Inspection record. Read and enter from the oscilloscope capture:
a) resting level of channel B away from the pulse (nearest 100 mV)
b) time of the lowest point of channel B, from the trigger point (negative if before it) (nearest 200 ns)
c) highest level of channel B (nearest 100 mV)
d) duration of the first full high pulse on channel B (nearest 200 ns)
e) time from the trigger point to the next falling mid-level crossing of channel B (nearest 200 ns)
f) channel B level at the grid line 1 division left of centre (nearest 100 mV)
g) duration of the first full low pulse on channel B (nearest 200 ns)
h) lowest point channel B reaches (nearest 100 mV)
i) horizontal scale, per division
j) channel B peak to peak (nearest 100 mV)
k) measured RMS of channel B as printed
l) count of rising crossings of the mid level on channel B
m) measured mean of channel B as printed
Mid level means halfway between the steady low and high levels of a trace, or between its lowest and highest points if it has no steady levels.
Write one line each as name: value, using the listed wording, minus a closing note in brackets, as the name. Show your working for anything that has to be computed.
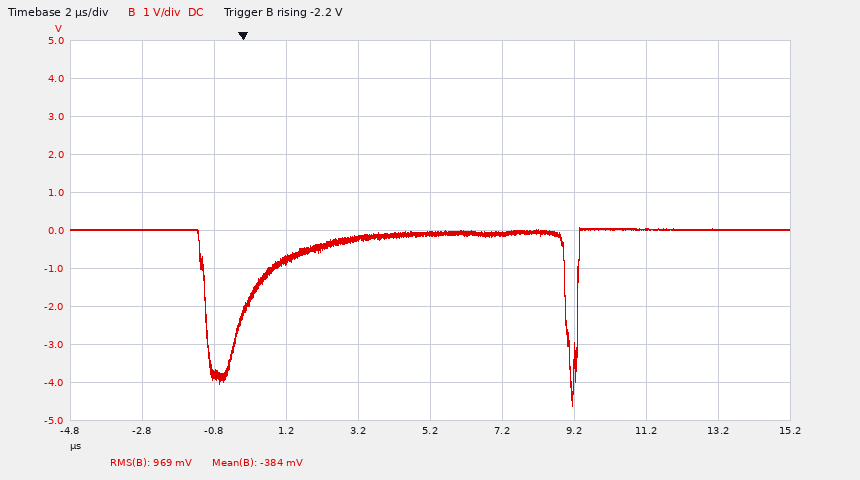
resting level of channel B away from the pulse: 0.0 V
time of the lowest point of channel B, from the trigger point (negative if before it): +9.2 µs
highest level of channel B: 100 mV
duration of the first full high pulse on channel B: 9.0 µs
time from the trigger point to the next falling mid-level crossing of channel B: 9.0 µs
channel B level at the grid line 1 division left of centre: -200 mV
duration of the first full low pulse on channel B: 1.0 µs
lowest point channel B reaches: -4.6 V
horizontal scale, per division: 2 µs
channel B peak to peak: 100 mV − (-4.6 V) = 4.7 V
measured RMS of channel B as printed: 969 mV
count of rising crossings of the mid level on channel B: 2
measured mean of channel B as printed: -384 mV
